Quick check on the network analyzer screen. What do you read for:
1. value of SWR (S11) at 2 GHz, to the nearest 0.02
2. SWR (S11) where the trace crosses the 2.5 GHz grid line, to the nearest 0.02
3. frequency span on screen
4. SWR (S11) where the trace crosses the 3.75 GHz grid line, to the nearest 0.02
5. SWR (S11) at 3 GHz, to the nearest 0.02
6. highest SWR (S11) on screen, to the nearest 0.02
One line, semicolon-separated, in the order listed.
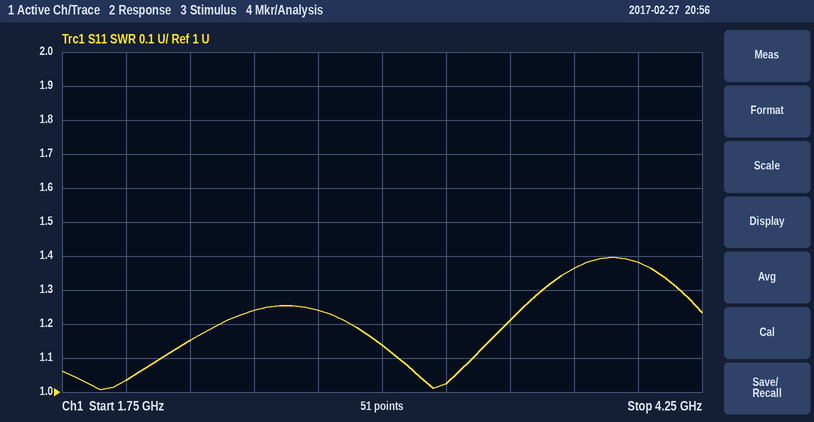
1.04; 1.24; 2.5 GHz; 1.36; 1.14; 1.40
